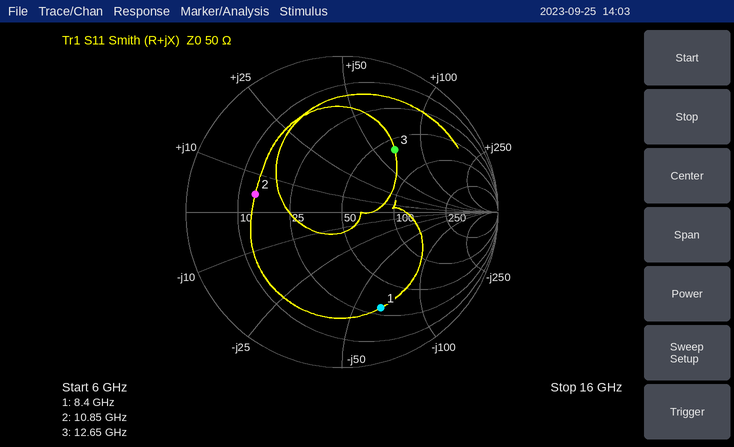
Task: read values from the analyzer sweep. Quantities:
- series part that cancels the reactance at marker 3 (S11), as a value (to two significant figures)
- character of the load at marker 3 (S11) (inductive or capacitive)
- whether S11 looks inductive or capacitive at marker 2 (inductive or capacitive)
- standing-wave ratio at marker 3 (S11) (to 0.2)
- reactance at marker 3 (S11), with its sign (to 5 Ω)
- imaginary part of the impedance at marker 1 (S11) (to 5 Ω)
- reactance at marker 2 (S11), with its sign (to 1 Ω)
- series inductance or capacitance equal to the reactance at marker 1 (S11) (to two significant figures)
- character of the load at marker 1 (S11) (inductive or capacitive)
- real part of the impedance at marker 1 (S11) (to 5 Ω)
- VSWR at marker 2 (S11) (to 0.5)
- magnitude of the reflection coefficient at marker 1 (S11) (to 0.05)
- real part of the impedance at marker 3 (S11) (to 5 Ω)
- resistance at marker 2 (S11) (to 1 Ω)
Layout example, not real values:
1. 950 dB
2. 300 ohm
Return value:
1. 190 fF
2. inductive
3. inductive
4. 3.2
5. +65 Ω
6. -65 Ω
7. +5 Ω
8. 290 fF
9. capacitive
10. 30 Ω
11. 3.5
12. 0.65
13. 60 Ω
14. 14 Ω
